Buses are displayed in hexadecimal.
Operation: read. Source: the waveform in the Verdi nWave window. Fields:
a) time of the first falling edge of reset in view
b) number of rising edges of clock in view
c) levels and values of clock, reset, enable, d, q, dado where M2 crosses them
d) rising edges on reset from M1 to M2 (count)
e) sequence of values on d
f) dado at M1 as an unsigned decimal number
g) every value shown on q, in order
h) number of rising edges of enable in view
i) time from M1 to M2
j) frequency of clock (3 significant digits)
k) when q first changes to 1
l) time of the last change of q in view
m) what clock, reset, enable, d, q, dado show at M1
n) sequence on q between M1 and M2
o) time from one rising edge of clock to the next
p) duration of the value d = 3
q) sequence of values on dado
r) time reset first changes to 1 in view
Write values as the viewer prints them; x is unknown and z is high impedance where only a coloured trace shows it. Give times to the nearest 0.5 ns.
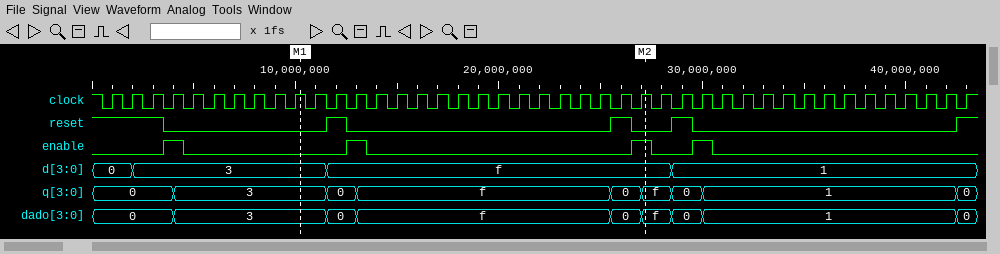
3.5 ns
43
clock=1, reset=0, enable=1, d=f, q=f, dado=f
2
0, 3, f, 1
3
0, 3, 0, f, 0, f, 0, 1, 0
4
17 ns
1.00 GHz
30 ns
42.5 ns
clock=1, reset=0, enable=0, d=3, q=3, dado=3
3, 0, f, 0, f
1 ns
9.5 ns
0, 3, 0, f, 0, f, 0, 1, 0
11.5 ns
